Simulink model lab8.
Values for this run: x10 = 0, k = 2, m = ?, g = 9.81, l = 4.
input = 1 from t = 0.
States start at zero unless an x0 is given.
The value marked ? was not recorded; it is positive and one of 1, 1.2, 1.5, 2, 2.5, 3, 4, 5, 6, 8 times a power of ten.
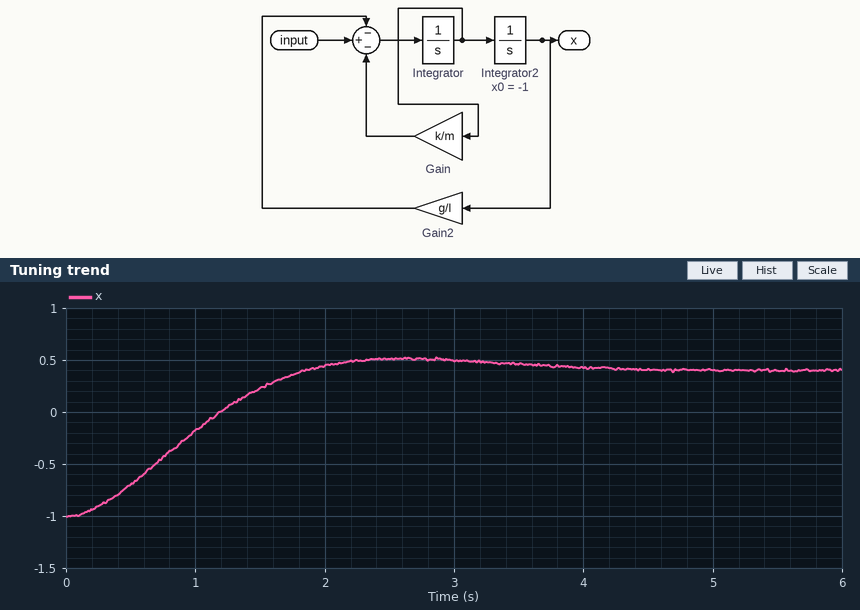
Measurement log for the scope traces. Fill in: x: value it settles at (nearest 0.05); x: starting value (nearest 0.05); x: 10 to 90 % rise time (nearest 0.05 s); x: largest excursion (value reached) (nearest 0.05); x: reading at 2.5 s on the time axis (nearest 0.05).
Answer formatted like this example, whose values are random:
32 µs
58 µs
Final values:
0.40
-1.00
1.25 s
0.50
0.50
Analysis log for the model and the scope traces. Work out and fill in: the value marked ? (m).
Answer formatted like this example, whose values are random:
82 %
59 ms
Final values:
1
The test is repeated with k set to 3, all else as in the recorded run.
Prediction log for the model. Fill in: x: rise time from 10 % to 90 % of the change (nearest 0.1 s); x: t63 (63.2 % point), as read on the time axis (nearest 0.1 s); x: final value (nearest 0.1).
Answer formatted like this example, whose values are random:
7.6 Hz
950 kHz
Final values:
2.0 s
1.3 s
0.4
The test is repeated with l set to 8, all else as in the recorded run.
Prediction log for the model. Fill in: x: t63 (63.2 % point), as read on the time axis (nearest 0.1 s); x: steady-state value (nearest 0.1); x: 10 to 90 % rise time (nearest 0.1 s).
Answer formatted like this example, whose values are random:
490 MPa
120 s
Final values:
1.8 s
0.8
2.6 s
